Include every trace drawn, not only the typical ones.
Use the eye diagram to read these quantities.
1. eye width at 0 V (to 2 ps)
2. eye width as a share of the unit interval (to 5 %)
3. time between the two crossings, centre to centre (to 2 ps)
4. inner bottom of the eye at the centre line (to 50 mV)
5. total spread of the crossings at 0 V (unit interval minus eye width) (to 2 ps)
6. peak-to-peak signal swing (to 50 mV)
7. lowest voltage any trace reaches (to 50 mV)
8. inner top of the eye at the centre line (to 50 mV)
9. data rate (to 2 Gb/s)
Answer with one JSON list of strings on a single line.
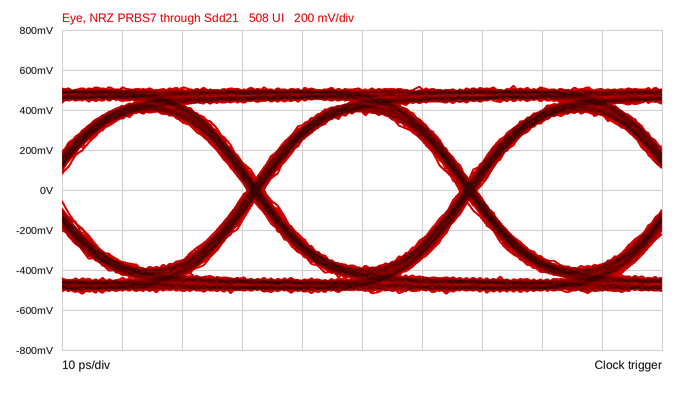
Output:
["32 ps", "90 %", "36 ps", "-400 mV", "4 ps", "1.05 V", "-500 mV", "400 mV", "28 Gb/s"]
